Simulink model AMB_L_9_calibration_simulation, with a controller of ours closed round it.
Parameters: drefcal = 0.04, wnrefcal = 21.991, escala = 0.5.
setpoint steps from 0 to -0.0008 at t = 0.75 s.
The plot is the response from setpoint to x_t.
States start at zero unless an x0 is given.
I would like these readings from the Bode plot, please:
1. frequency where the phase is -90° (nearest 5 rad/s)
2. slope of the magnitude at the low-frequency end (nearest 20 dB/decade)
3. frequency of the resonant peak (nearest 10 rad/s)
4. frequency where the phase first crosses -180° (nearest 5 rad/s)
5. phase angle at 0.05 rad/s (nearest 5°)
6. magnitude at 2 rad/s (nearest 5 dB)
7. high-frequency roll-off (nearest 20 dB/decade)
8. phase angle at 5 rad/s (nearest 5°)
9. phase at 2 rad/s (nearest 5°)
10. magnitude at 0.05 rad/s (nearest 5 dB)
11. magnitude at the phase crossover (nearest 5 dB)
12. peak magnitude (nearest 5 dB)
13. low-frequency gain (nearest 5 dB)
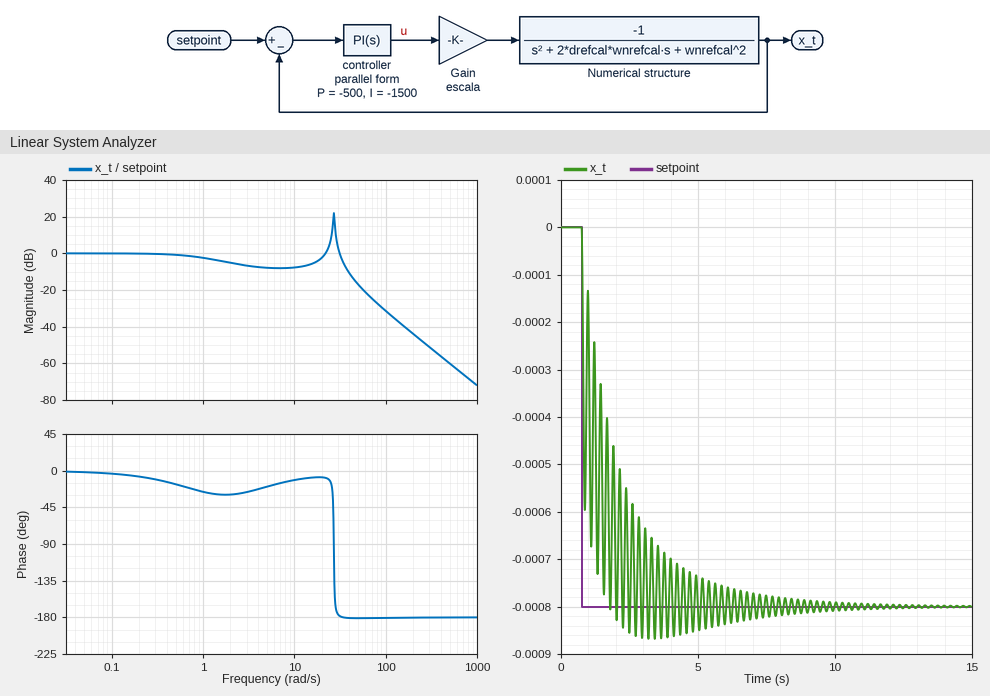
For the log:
25 rad/s
0 dB/decade
30 rad/s
35 rad/s
0°
-5 dB
-40 dB/decade
-20°
-30°
0 dB
-5 dB
20 dB
0 dB
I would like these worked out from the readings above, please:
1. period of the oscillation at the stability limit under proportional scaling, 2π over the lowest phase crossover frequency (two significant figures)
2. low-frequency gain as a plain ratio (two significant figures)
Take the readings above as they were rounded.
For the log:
0.18 s
1.0
